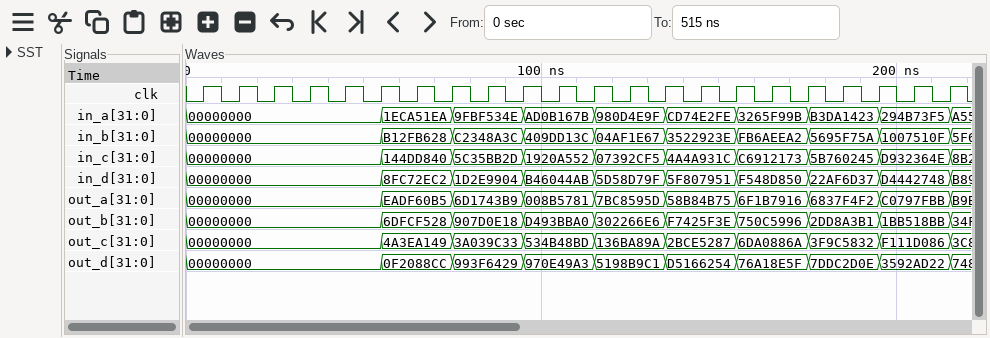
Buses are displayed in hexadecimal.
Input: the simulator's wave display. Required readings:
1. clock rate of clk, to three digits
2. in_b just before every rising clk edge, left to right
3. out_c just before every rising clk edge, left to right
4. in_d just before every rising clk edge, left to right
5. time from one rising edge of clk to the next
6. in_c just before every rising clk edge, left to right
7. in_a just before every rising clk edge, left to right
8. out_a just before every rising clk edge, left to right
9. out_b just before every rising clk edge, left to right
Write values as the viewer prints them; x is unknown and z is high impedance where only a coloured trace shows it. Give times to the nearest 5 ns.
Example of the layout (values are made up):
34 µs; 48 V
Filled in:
100 MHz; 00000000, 00000000, 00000000, 00000000, 00000000, 00000000, B12FB628, B12FB628, C2348A3C, C2348A3C, 409DD13C, 409DD13C, 04AF1E67, 04AF1E67, 3522923E, 3522923E, FB6AEEA2, FB6AEEA2, 5695F75A, 5695F75A, 1007510F, 1007510F; 00000000, 00000000, 00000000, 00000000, 00000000, 00000000, 4A3EA149, 4A3EA149, 3A039C33, 3A039C33, 534B48BD, 534B48BD, 136BA89A, 136BA89A, 2BCE5287, 2BCE5287, 6DA0886A, 6DA0886A, 3F9C5832, 3F9C5832, F111D086, F111D086; 00000000, 00000000, 00000000, 00000000, 00000000, 00000000, 8FC72EC2, 8FC72EC2, 1D2E9904, 1D2E9904, B46044AB, B46044AB, 5D58D79F, 5D58D79F, 5F807951, 5F807951, F548D850, F548D850, 22AF6D37, 22AF6D37, D4442748, D4442748; 10 ns; 00000000, 00000000, 00000000, 00000000, 00000000, 00000000, 144DD840, 144DD840, 5C35BB2D, 5C35BB2D, 1920A552, 1920A552, 07392CF5, 07392CF5, 4A4A931C, 4A4A931C, C6912173, C6912173, 5B760245, 5B760245, D932364E, D932364E; 00000000, 00000000, 00000000, 00000000, 00000000, 00000000, 1ECA51EA, 1ECA51EA, 9FBF534E, 9FBF534E, AD0B167B, AD0B167B, 980D4E9F, 980D4E9F, CD74E2FE, CD74E2FE, 3265F99B, 3265F99B, B3DA1423, B3DA1423, 294B73F5, 294B73F5; 00000000, 00000000, 00000000, 00000000, 00000000, 00000000, EADF60B5, EADF60B5, 6D1743B9, 6D1743B9, 008B5781, 008B5781, 7BC8595D, 7BC8595D, 58B84B75, 58B84B75, 6F1B7916, 6F1B7916, 6837F4F2, 6837F4F2, C0797FBB, C0797FBB; 00000000, 00000000, 00000000, 00000000, 00000000, 00000000, 6DFCF528, 6DFCF528, 907D0E18, 907D0E18, D493BBA0, D493BBA0, 302266E6, 302266E6, F7425F3E, F7425F3E, 750C5996, 750C5996, 2DD8A3B1, 2DD8A3B1, 1BB518BB, 1BB518BB
